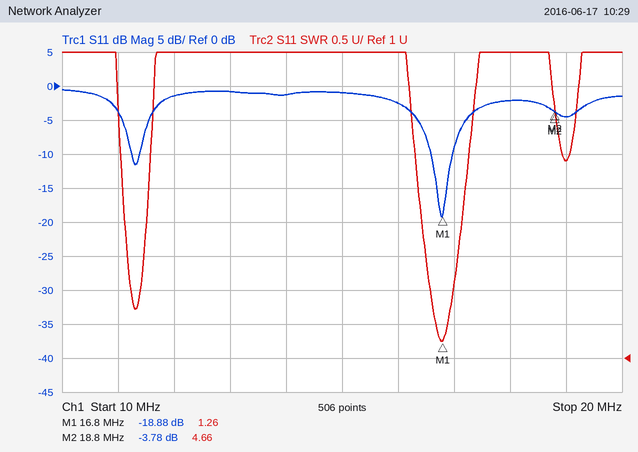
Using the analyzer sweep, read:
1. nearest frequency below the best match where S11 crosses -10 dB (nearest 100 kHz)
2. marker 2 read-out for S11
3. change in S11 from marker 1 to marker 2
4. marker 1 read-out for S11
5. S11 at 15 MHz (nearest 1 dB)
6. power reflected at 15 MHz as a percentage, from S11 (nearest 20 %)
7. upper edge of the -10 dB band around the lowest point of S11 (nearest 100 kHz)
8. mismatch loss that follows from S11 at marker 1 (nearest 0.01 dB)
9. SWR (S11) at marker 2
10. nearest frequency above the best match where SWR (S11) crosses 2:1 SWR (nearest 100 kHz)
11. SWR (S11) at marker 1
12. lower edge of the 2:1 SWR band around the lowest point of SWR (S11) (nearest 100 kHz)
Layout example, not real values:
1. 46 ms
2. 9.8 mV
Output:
1. 16.6 MHz
2. -3.78 dB
3. 15.10 dB
4. -18.88 dB
5. -1 dB
6. 80 %
7. 17.0 MHz
8. 0.06 dB
9. 4.66
10. 17.0 MHz
11. 1.26
12. 16.6 MHz
